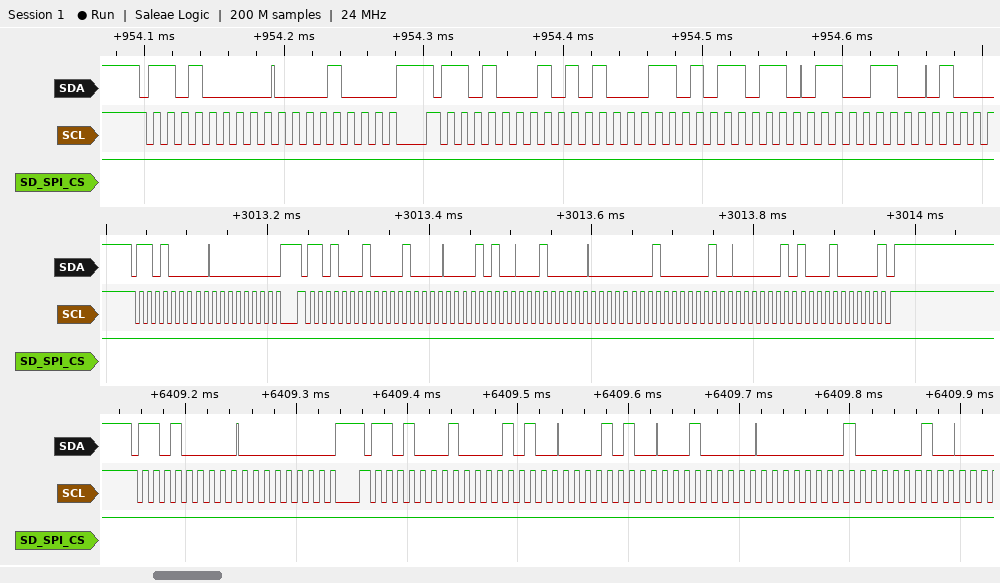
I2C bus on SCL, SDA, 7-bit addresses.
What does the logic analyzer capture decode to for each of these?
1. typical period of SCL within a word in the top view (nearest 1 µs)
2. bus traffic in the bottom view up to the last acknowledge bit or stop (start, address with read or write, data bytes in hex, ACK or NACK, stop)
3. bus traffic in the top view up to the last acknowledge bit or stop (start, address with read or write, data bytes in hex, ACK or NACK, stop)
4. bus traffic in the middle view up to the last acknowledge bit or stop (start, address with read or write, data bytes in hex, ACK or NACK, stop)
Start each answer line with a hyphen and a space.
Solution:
- 10 µs
- start, address 68 write ACK, 00 ACK, repeated start, address 68 read ACK, 14 ACK, 14 ACK, 20 ACK, 01 ACK, 04 ACK
- start, address 68 write ACK, 08 ACK, repeated start, address 68 read ACK, A3 ACK, B6 ACK, CC ACK
- start, address 68 write ACK, 00 ACK, repeated start, address 68 read ACK, 10 ACK, 14 ACK, 20 ACK, 01 ACK, 04 ACK, 05 ACK, 20 NACK, stop
